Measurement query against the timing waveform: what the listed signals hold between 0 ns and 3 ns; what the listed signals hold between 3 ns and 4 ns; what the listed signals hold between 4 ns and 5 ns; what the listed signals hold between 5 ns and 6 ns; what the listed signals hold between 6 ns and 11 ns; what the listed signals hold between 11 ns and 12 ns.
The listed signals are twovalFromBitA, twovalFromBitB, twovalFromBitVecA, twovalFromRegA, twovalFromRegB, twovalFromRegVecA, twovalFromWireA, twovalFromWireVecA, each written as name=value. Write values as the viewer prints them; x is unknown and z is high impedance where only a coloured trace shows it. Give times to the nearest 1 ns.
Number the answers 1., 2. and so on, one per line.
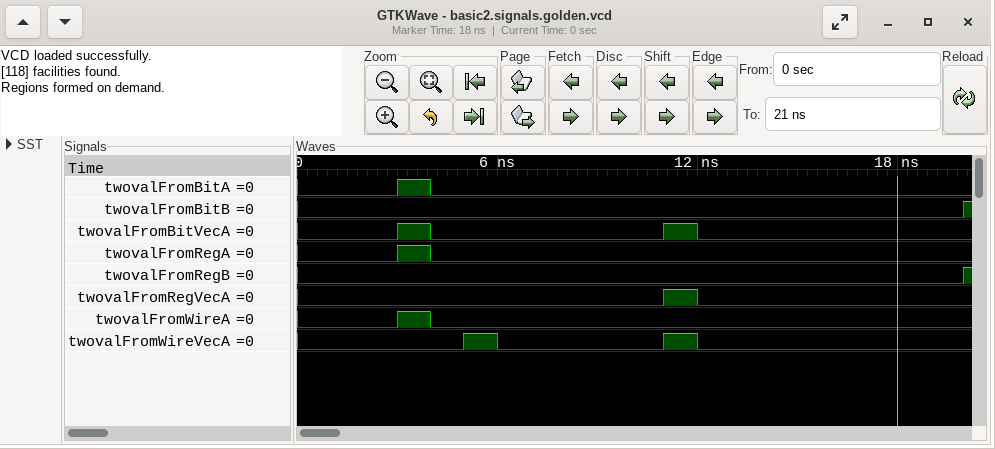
1. twovalFromBitA=0, twovalFromBitB=0, twovalFromBitVecA=0, twovalFromRegA=0, twovalFromRegB=0, twovalFromRegVecA=0, twovalFromWireA=0, twovalFromWireVecA=0
2. twovalFromBitA=1, twovalFromBitB=0, twovalFromBitVecA=1, twovalFromRegA=1, twovalFromRegB=0, twovalFromRegVecA=0, twovalFromWireA=1, twovalFromWireVecA=0
3. twovalFromBitA=0, twovalFromBitB=0, twovalFromBitVecA=0, twovalFromRegA=0, twovalFromRegB=0, twovalFromRegVecA=0, twovalFromWireA=0, twovalFromWireVecA=0
4. twovalFromBitA=0, twovalFromBitB=0, twovalFromBitVecA=0, twovalFromRegA=0, twovalFromRegB=0, twovalFromRegVecA=0, twovalFromWireA=0, twovalFromWireVecA=1
5. twovalFromBitA=0, twovalFromBitB=0, twovalFromBitVecA=0, twovalFromRegA=0, twovalFromRegB=0, twovalFromRegVecA=0, twovalFromWireA=0, twovalFromWireVecA=0
6. twovalFromBitA=0, twovalFromBitB=0, twovalFromBitVecA=1, twovalFromRegA=0, twovalFromRegB=0, twovalFromRegVecA=1, twovalFromWireA=0, twovalFromWireVecA=1
